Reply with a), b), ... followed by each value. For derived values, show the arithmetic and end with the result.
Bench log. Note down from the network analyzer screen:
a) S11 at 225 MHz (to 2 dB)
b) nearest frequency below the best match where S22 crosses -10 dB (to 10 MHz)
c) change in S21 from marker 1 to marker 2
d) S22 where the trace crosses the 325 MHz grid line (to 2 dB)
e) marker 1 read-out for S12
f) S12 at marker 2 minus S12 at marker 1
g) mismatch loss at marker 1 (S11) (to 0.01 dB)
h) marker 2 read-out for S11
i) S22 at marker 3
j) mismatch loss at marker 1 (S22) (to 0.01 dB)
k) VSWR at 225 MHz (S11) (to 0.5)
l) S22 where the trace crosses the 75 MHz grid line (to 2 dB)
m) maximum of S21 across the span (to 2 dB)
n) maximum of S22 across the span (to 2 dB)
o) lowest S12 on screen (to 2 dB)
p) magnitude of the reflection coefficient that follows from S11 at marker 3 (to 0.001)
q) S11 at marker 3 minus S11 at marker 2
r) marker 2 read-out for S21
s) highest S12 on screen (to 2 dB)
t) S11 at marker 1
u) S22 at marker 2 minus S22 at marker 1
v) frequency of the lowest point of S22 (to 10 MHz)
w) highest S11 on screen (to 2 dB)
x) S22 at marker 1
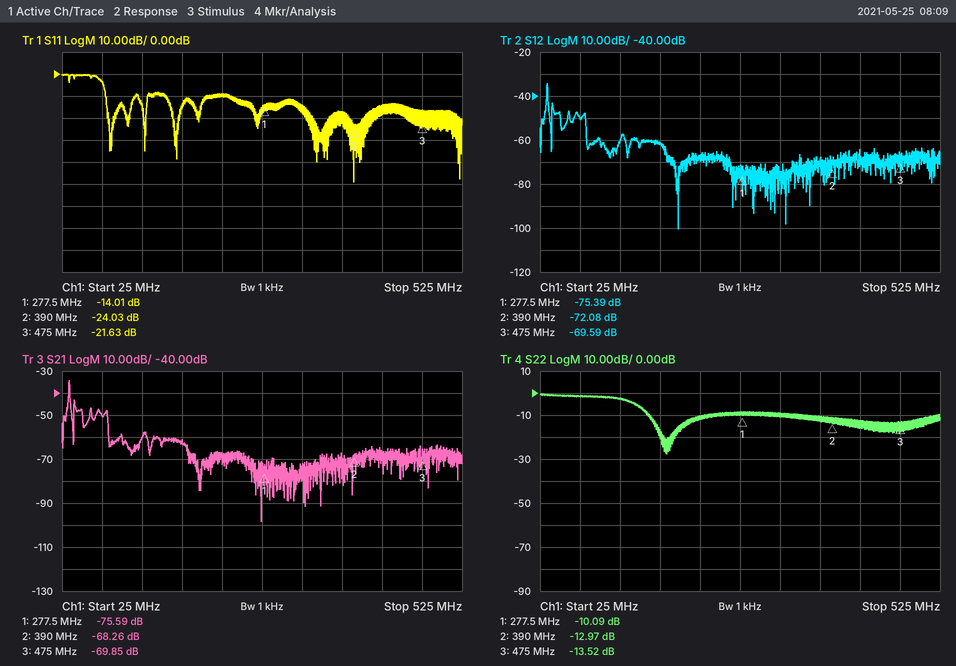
a) -10 dB
b) 160 MHz
c) -68.26 − (-75.59) = 7.33 dB
d) -10 dB
e) -75.39 dB
f) -72.08 − (-75.39) = 3.31 dB
g) −10 log10(1 − 10^(-14.01/10)) ≈ 0.18 dB
h) -24.03 dB
i) -13.52 dB
j) −10 log10(1 − 10^(-10.09/10)) ≈ 0.45 dB
k) |Γ| = 10^(-10/20) = 0.3162; VSWR = (1 + 0.3162)/(1 − 0.3162) ≈ 1.92, so 2.0 to the nearest 0.5
l) -2 dB
m) -34 dB
n) 0 dB
o) -100 dB
p) 10^(-21.63/20) ≈ 0.083
q) -21.63 − (-24.03) = 2.40 dB
r) -68.26 dB
s) -34 dB
t) -14.01 dB
u) -12.97 − (-10.09) = -2.88 dB
v) 180 MHz
w) 0 dB
x) -10.09 dB
